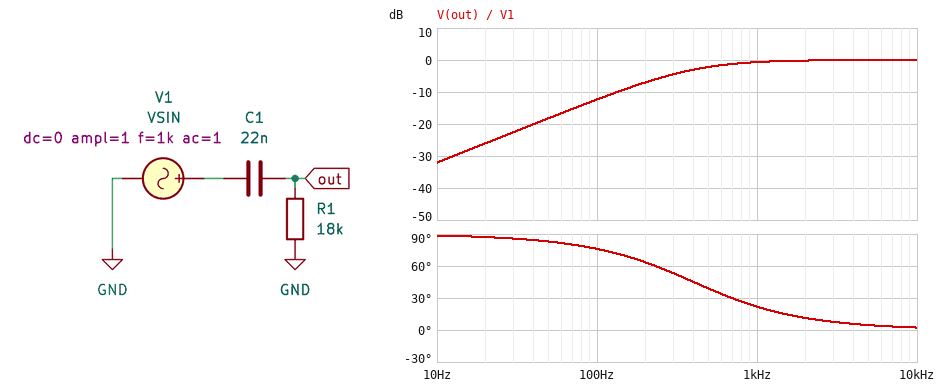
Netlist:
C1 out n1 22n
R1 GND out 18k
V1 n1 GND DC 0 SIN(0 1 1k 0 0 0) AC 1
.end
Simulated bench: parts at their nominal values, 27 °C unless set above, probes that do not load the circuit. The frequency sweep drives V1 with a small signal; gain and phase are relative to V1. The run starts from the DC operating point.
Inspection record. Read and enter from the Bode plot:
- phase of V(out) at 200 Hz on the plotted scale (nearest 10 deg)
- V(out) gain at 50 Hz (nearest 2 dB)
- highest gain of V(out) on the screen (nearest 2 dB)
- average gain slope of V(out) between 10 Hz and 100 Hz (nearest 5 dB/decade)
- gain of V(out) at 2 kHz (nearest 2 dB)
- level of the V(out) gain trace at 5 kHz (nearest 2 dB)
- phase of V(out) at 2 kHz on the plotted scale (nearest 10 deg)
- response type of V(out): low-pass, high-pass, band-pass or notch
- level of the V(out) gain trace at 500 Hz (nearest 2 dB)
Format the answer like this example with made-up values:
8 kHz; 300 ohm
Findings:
60 deg; -18 dB; 0 dB; 20 dB/decade; 0 dB; 0 dB; 10 deg; high-pass; -2 dB
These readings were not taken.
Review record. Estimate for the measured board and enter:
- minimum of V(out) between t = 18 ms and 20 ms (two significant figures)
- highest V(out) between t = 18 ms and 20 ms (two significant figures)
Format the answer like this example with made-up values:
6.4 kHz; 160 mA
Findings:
-930 mV; 930 mV
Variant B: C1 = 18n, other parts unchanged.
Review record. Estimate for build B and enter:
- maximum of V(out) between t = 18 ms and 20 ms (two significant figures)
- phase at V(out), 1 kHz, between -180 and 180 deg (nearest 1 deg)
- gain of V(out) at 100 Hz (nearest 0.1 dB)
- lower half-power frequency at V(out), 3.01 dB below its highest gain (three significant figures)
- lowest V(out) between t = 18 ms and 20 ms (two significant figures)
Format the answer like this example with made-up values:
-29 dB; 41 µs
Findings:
900 mV; 26 deg; -14.0 dB; 491 Hz; -900 mV
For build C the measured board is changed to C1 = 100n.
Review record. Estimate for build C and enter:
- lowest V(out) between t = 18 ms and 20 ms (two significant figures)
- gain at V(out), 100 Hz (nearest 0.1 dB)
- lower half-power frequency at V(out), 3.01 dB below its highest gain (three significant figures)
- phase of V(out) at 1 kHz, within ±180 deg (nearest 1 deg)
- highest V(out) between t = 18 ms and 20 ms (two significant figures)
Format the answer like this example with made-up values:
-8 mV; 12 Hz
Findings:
-1.0 V; -2.5 dB; 88.4 Hz; 5 deg; 1.0 V
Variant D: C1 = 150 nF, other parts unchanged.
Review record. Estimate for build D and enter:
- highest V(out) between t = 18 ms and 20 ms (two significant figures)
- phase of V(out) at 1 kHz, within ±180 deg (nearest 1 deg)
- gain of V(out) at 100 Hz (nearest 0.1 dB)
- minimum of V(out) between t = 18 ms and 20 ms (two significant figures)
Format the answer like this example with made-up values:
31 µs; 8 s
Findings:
1.0 V; 3 deg; -1.3 dB; -1.0 V
